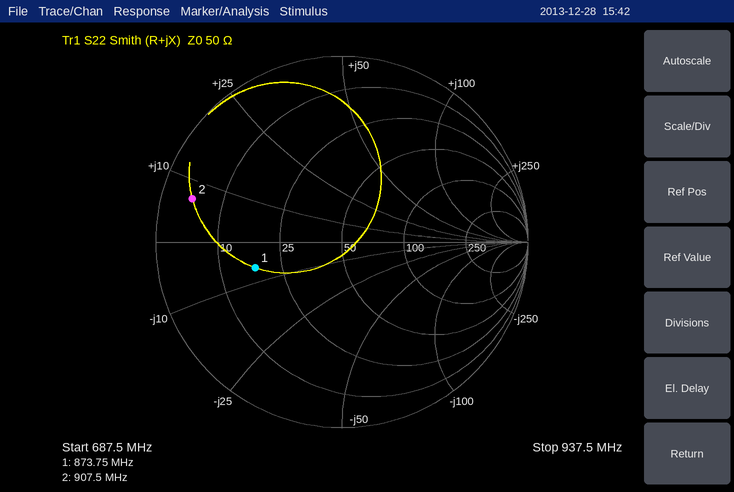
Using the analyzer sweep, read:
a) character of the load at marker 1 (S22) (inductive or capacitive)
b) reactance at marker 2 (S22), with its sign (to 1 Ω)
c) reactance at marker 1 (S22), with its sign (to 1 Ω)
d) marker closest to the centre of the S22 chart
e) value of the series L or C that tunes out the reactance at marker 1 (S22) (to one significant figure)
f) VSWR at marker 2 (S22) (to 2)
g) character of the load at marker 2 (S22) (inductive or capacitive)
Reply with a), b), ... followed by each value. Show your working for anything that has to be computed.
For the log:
a) capacitive
b) +7 Ω
c) -6 Ω
d) marker 1
e) L = 6 Ω/(2π × 873.75 MHz) ≈ 1 nH
f) 12
g) inductive
